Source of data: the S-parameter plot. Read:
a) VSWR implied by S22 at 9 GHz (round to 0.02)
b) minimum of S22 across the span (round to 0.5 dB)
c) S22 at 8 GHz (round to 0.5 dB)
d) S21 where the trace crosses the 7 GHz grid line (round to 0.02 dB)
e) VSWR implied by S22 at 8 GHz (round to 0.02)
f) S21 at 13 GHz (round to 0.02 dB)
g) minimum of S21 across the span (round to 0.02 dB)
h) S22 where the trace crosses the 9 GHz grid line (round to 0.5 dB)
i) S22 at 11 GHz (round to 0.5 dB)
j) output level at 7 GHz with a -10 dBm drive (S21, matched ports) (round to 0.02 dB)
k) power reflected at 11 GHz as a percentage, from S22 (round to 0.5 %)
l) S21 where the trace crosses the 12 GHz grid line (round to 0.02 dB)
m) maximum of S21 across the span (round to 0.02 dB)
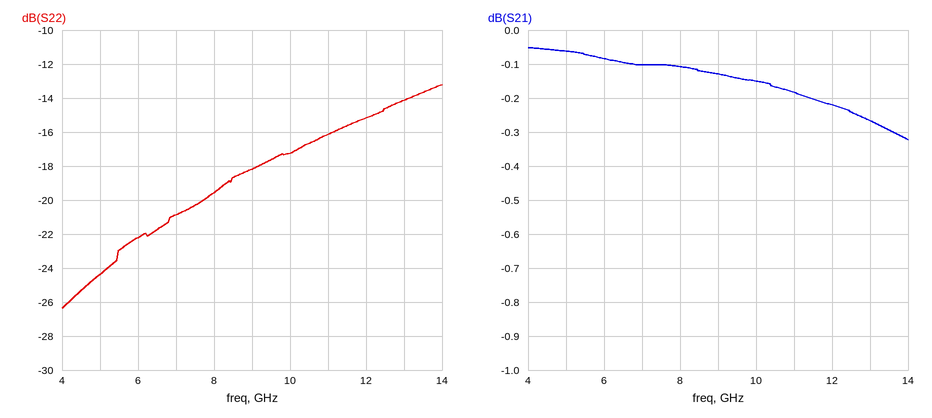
1.28
-26.5 dB
-19.5 dB
-0.10 dB
1.24
-0.26 dB
-0.32 dB
-18.0 dB
-16.0 dB
-10.10 dBm
2.5 %
-0.22 dB
-0.06 dB
